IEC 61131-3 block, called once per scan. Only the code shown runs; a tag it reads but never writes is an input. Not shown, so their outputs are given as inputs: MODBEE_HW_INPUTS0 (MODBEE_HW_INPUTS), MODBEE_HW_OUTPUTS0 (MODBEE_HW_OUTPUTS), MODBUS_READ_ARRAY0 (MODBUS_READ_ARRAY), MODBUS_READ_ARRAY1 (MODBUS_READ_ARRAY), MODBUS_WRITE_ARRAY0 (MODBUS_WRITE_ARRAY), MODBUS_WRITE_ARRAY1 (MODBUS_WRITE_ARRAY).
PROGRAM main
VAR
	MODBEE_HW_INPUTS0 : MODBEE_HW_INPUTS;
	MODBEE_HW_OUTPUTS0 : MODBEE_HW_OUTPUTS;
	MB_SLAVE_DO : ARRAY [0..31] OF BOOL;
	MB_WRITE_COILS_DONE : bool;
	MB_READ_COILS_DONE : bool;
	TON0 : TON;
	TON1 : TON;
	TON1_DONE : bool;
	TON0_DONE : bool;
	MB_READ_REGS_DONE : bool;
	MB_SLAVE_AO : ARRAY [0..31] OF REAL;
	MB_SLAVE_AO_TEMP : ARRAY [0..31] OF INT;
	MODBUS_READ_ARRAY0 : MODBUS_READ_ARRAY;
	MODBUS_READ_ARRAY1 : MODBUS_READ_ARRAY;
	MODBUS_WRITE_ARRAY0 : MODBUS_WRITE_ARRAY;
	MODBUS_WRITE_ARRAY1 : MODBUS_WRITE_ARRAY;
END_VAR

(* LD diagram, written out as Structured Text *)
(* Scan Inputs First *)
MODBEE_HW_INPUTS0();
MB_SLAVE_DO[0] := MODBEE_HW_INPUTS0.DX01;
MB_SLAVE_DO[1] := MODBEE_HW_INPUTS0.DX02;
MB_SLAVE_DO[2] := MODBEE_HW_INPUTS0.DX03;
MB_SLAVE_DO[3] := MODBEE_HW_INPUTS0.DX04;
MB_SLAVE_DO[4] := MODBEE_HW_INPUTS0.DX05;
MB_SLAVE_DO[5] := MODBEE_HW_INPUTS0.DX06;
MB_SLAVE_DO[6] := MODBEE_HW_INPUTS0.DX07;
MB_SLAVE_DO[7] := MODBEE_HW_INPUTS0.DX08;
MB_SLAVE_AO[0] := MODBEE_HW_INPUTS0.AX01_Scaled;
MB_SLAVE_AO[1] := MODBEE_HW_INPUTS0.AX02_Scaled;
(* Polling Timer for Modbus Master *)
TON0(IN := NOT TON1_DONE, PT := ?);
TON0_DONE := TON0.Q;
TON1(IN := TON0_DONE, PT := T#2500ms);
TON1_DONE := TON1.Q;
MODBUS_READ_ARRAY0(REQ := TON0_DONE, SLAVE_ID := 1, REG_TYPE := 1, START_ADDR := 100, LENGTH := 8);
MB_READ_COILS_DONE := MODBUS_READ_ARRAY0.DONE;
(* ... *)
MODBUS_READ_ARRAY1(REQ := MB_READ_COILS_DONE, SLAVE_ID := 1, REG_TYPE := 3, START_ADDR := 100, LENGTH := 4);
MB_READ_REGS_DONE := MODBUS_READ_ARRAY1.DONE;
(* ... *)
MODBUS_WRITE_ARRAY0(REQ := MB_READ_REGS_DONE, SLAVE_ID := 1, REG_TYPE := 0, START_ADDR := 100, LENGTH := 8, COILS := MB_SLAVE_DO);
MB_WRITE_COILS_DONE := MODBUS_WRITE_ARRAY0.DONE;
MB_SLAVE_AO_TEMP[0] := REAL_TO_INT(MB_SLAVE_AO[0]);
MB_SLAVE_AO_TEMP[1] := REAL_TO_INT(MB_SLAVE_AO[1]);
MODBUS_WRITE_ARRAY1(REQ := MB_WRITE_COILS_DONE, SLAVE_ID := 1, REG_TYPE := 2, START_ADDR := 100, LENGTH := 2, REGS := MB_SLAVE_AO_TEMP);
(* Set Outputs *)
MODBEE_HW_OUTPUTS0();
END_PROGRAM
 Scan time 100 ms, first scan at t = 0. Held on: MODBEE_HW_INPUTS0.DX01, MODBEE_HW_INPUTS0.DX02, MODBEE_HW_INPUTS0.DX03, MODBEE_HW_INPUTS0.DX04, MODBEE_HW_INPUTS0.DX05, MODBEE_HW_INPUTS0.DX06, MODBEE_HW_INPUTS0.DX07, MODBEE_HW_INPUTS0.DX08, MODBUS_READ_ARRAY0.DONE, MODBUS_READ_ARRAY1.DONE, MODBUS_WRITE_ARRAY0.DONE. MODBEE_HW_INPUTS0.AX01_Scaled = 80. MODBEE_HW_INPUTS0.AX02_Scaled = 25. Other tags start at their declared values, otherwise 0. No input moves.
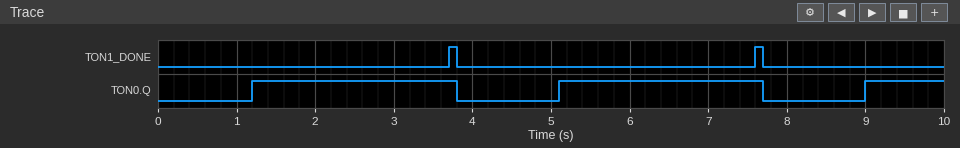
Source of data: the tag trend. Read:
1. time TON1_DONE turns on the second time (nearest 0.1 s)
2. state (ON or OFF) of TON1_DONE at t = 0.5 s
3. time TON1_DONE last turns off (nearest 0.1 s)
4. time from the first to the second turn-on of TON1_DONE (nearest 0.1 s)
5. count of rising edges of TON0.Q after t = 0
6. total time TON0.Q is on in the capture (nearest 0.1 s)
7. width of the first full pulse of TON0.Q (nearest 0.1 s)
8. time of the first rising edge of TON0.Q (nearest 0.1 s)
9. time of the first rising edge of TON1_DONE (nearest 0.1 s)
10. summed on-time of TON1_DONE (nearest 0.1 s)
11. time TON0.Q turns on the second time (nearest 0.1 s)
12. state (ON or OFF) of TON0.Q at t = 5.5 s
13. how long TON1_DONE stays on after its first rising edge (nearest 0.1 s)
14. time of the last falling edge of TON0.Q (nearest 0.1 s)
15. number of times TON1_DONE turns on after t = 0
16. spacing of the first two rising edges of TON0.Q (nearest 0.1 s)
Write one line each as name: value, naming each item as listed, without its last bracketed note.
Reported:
time TON1_DONE turns on the second time: 7.6 s
state (ON or OFF) of TON1_DONE at t = 0.5 s: OFF
time TON1_DONE last turns off: 7.7 s
time from the first to the second turn-on of TON1_DONE: 3.9 s
count of rising edges of TON0.Q after t = 0: 3
total time TON0.Q is on in the capture: 6.2 s
width of the first full pulse of TON0.Q: 2.6 s
time of the first rising edge of TON0.Q: 1.2 s
time of the first rising edge of TON1_DONE: 3.7 s
summed on-time of TON1_DONE: 0.2 s
time TON0.Q turns on the second time: 5.1 s
state (ON or OFF) of TON0.Q at t = 5.5 s: ON
how long TON1_DONE stays on after its first rising edge: 0.1 s
time of the last falling edge of TON0.Q: 7.7 s
number of times TON1_DONE turns on after t = 0: 2
spacing of the first two rising edges of TON0.Q: 3.9 s
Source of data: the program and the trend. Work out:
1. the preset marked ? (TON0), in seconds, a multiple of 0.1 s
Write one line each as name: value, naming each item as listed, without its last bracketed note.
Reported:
the preset marked ? (TON0), in seconds, a multiple of 0.1 s: 1.2 s
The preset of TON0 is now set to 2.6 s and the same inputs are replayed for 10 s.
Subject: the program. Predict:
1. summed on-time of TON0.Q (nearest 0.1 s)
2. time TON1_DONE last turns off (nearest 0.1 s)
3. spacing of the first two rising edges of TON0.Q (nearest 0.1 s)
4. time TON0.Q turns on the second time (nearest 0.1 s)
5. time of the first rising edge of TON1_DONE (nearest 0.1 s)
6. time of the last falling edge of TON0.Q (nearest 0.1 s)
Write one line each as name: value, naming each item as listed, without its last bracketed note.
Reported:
summed on-time of TON0.Q: 4.7 s
time TON1_DONE last turns off: 5.2 s
spacing of the first two rising edges of TON0.Q: 5.3 s
time TON0.Q turns on the second time: 7.9 s
time of the first rising edge of TON1_DONE: 5.1 s
time of the last falling edge of TON0.Q: 5.2 s
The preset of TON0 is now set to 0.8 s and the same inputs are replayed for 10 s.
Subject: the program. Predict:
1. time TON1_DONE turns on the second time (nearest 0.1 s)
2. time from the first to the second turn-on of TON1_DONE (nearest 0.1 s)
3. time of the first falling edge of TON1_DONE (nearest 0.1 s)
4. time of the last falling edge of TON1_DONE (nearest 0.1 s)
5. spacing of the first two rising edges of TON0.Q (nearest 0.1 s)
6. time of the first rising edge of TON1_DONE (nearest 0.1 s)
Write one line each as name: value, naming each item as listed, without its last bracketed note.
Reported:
time TON1_DONE turns on the second time: 6.8 s
time from the first to the second turn-on of TON1_DONE: 3.5 s
time of the first falling edge of TON1_DONE: 3.4 s
time of the last falling edge of TON1_DONE: 6.9 s
spacing of the first two rising edges of TON0.Q: 3.5 s
time of the first rising edge of TON1_DONE: 3.3 s
